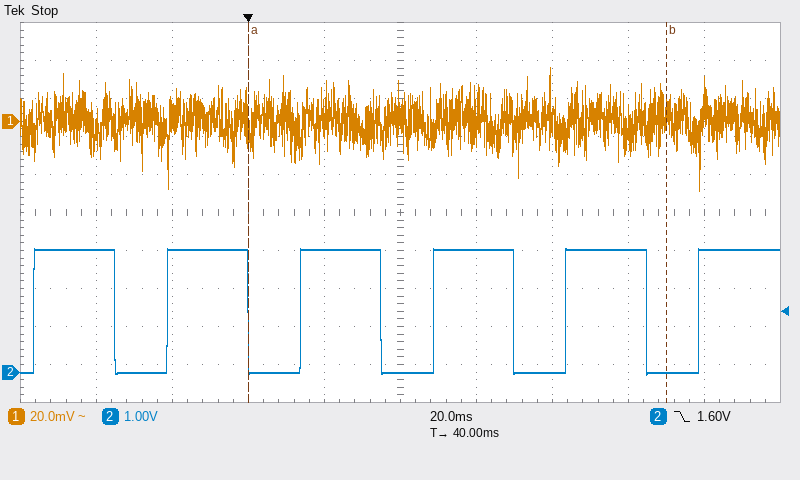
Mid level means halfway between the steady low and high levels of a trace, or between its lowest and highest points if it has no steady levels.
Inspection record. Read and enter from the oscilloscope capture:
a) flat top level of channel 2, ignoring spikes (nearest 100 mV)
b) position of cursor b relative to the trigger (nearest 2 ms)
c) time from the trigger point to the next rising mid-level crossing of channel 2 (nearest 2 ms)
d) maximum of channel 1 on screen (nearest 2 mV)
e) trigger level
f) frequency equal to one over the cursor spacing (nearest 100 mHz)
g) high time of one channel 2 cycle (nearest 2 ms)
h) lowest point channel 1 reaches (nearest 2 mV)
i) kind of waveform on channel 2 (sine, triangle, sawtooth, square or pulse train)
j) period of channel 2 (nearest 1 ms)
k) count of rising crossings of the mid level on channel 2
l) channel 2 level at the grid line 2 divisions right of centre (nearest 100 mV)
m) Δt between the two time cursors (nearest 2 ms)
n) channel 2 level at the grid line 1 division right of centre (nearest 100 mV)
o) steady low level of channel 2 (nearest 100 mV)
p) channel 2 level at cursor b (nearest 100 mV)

3.2 V
+110 ms
14 ms
28 mV
1.60 V
9.1 Hz
22 ms
-36 mV
pulse train
35 ms
6
0.0 V
110 ms
3.2 V
0.0 V
0.0 V
